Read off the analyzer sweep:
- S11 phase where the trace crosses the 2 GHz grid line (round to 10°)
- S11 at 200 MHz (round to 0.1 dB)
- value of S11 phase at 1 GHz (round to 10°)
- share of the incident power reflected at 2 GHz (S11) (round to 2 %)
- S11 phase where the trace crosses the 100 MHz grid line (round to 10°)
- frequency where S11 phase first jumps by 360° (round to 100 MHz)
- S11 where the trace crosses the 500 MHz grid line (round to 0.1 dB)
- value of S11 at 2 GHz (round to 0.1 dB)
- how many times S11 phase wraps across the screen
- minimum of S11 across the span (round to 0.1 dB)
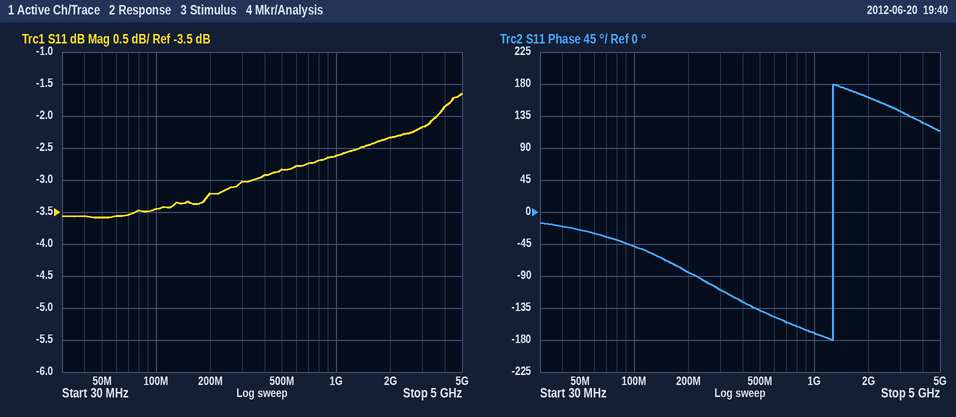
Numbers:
160°
-3.2 dB
-170°
58 %
-50°
1.3 GHz
-2.8 dB
-2.3 dB
1
-3.6 dB
